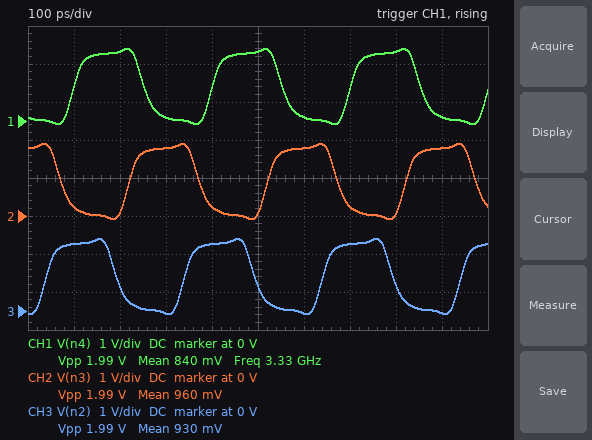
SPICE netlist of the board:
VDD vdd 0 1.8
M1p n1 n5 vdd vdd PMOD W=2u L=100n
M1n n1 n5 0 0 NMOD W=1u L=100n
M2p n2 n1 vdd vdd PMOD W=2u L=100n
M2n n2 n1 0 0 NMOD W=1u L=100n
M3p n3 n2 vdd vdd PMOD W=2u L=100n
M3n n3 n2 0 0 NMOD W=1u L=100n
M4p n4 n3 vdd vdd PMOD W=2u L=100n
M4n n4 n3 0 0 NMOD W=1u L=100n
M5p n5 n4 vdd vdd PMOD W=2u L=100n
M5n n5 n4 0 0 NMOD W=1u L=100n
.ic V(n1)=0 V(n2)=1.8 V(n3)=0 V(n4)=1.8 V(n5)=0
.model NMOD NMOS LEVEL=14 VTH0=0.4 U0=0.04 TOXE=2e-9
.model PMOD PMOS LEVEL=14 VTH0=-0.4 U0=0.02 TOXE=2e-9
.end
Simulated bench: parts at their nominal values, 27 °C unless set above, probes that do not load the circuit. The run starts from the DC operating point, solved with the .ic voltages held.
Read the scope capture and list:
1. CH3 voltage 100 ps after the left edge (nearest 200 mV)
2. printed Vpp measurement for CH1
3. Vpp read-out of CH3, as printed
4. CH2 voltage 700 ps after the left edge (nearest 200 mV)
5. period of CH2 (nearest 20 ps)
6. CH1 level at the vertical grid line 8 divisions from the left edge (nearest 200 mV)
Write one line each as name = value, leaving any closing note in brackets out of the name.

CH3 voltage 100 ps after the left edge = 1.8 V
printed Vpp measurement for CH1 = 1.99 V
Vpp read-out of CH3, as printed = 1.99 V
CH2 voltage 700 ps after the left edge = 200 mV
period of CH2 = 300 ps
CH1 level at the vertical grid line 8 divisions from the left edge = 1.8 V
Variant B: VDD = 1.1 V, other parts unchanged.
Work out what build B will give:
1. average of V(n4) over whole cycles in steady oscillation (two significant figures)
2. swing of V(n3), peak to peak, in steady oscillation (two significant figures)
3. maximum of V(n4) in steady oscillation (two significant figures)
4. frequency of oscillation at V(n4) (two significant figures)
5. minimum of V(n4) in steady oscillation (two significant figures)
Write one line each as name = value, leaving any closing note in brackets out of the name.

average of V(n4) over whole cycles in steady oscillation = 560 mV
swing of V(n3), peak to peak, in steady oscillation = 1.3 V
maximum of V(n4) in steady oscillation = 1.2 V
frequency of oscillation at V(n4) = 1.5 GHz
minimum of V(n4) in steady oscillation = -110 mV
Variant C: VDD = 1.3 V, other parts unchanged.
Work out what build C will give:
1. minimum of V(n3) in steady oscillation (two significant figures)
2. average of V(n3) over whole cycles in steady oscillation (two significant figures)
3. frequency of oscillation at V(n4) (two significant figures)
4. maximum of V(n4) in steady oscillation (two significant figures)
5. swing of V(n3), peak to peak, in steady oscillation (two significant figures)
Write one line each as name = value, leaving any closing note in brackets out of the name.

minimum of V(n3) in steady oscillation = -96 mV
average of V(n3) over whole cycles in steady oscillation = 660 mV
frequency of oscillation at V(n4) = 2.1 GHz
maximum of V(n4) in steady oscillation = 1.4 V
swing of V(n3), peak to peak, in steady oscillation = 1.5 V
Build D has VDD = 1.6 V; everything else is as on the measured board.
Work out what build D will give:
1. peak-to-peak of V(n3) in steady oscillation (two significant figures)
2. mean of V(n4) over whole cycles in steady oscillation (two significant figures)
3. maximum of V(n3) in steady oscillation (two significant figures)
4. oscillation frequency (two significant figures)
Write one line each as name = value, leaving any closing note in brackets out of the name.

peak-to-peak of V(n3) in steady oscillation = 1.8 V
mean of V(n4) over whole cycles in steady oscillation = 820 mV
maximum of V(n3) in steady oscillation = 1.7 V
oscillation frequency = 2.9 GHz
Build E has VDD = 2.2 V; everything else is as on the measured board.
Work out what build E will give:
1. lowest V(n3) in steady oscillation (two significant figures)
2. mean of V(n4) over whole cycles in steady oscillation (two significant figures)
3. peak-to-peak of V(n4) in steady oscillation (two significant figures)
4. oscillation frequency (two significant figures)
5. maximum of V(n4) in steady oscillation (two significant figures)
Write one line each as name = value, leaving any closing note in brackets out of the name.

lowest V(n3) in steady oscillation = -86 mV
mean of V(n4) over whole cycles in steady oscillation = 1.1 V
peak-to-peak of V(n4) in steady oscillation = 2.4 V
oscillation frequency = 4.1 GHz
maximum of V(n4) in steady oscillation = 2.3 V
